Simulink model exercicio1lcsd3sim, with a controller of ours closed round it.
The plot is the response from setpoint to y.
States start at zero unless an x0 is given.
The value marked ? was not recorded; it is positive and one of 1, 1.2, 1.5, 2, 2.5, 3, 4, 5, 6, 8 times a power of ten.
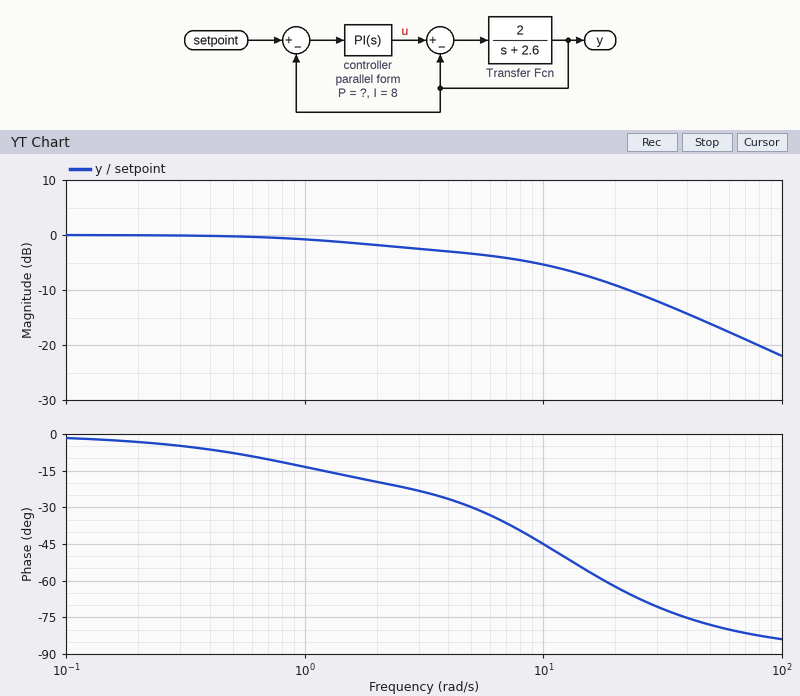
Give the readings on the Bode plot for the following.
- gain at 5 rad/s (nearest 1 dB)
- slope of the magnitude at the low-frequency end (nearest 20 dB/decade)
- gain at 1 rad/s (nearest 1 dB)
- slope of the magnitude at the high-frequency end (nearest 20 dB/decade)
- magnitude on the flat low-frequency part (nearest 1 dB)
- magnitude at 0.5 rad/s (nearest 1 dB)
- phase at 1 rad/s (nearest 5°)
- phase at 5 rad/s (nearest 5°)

-3 dB
0 dB/decade
-1 dB
-20 dB/decade
0 dB
0 dB
-15°
-30°
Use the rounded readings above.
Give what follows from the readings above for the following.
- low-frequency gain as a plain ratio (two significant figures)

1.0
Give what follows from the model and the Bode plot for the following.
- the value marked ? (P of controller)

4
